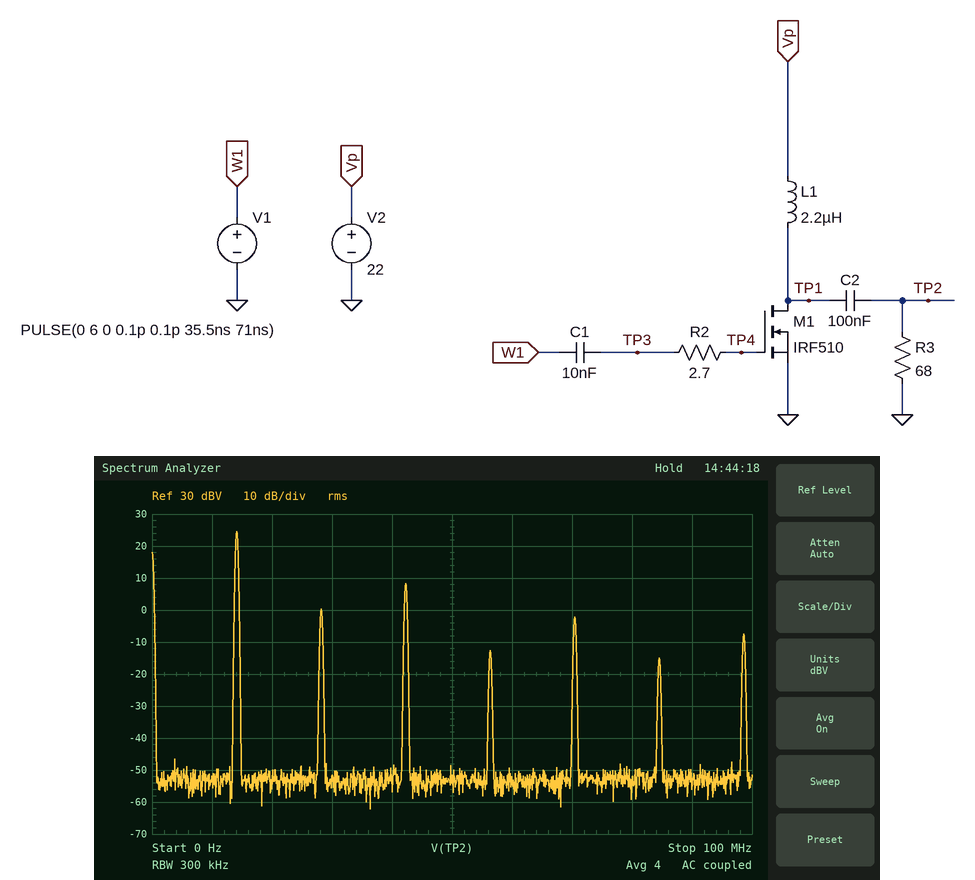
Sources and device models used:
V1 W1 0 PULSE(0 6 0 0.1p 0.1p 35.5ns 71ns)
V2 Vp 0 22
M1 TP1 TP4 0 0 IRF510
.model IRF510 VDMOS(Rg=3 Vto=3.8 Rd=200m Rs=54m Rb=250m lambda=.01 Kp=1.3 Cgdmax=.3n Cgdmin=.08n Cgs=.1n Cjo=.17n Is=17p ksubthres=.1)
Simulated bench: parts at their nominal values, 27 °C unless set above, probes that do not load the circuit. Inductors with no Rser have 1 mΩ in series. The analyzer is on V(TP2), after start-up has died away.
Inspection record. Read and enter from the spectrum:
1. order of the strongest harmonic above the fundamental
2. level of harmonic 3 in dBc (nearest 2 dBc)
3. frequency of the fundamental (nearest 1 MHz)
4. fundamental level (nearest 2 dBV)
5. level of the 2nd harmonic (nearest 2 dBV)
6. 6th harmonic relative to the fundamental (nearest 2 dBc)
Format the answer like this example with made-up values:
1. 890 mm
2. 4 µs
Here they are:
1. 3
2. -16 dBc
3. 14 MHz
4. 24 dBV
5. 0 dBV
6. -40 dBc
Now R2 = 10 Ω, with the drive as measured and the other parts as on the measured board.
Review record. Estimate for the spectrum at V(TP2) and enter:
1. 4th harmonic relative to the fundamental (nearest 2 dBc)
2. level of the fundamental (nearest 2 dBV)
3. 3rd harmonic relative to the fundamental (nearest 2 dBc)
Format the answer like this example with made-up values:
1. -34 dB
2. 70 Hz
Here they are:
1. -30 dBc
2. 22 dBV
3. -18 dBc
